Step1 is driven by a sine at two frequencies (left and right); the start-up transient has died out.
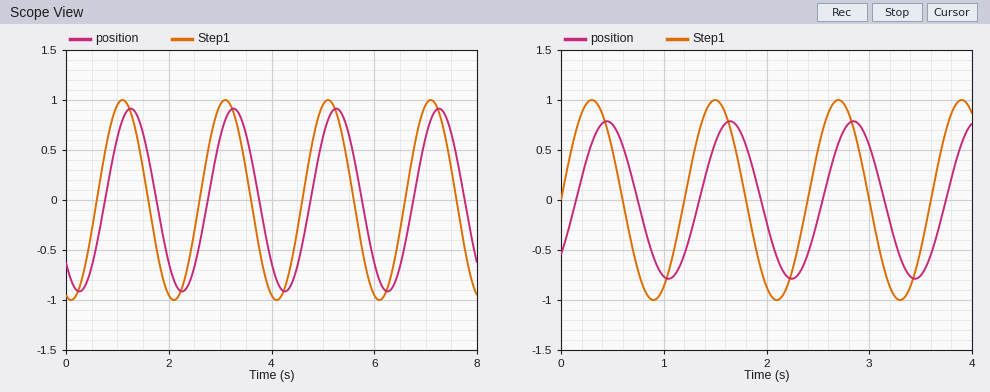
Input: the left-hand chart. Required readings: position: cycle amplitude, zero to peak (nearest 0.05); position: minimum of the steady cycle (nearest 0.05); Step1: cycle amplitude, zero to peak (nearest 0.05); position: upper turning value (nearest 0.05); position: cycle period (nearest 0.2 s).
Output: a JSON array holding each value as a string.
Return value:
["0.90", "-0.90", "1.00", "0.90", "2.0 s"]
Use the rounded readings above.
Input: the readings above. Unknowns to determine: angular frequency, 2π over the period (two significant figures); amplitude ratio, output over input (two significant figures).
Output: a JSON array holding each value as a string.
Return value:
["3.1 rad/s", "0.90"]
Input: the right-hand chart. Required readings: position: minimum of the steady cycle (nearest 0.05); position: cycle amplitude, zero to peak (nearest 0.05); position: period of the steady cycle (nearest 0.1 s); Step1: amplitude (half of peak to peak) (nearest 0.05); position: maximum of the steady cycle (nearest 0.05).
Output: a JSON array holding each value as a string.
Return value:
["-0.80", "0.80", "1.2 s", "1.00", "0.80"]
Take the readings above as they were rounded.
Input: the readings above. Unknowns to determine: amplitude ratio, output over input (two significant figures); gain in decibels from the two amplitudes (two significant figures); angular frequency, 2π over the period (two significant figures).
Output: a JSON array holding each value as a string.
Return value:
["0.80", "-1.9 dB", "5.2 rad/s"]
